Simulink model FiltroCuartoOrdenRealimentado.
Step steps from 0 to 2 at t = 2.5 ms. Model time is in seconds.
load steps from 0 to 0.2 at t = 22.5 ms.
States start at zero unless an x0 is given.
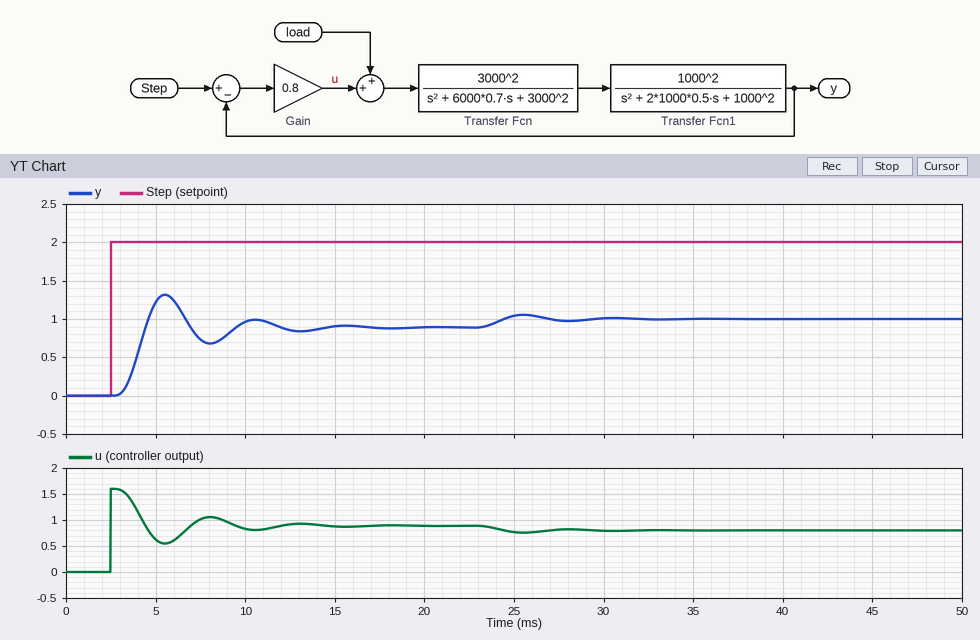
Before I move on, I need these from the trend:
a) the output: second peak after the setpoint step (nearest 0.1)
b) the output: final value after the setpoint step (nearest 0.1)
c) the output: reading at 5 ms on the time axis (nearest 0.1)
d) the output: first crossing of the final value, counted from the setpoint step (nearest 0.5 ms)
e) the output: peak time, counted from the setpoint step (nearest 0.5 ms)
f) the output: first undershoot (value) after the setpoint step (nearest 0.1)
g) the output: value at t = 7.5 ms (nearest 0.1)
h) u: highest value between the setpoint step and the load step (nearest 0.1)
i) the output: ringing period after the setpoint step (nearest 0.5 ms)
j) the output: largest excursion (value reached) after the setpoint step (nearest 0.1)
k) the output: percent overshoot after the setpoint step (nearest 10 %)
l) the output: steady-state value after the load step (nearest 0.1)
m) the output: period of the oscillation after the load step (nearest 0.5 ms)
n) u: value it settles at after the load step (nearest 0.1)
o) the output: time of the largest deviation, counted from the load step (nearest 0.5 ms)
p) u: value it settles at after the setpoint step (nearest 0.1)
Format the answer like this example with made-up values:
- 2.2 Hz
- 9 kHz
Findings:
- 1.0
- 0.9
- 1.2
- 2.0 ms
- 3.0 ms
- 0.7
- 0.7
- 1.6
- 5.0 ms
- 1.3
- 50 %
- 1.0
- 5.0 ms
- 0.8
- 3.0 ms
- 0.9
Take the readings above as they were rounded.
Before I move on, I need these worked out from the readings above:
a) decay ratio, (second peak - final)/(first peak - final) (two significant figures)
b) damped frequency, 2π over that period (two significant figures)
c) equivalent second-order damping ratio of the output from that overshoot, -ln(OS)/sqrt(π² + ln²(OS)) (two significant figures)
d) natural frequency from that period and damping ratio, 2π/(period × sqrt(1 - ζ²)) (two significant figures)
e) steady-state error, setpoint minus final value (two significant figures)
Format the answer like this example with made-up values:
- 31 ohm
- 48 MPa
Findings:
- 0.25
- 1.3 rad/ms
- 0.22
- 1.3 rad/ms
- 1.1
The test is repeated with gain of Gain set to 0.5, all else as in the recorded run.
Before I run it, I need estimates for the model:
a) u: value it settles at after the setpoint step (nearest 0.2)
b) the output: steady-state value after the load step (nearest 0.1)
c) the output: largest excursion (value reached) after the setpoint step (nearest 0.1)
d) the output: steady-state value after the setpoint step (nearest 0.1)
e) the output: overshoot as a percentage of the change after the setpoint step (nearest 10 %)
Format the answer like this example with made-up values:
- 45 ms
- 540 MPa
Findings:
- 0.6
- 0.8
- 0.9
- 0.7
- 40 %
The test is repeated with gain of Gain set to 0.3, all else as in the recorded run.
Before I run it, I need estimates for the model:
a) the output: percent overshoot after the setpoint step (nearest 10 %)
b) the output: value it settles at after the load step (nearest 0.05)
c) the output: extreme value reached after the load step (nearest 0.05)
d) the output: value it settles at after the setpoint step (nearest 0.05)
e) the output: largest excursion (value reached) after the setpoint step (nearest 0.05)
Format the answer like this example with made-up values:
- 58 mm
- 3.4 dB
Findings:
- 30 %
- 0.60
- 0.65
- 0.45
- 0.60
